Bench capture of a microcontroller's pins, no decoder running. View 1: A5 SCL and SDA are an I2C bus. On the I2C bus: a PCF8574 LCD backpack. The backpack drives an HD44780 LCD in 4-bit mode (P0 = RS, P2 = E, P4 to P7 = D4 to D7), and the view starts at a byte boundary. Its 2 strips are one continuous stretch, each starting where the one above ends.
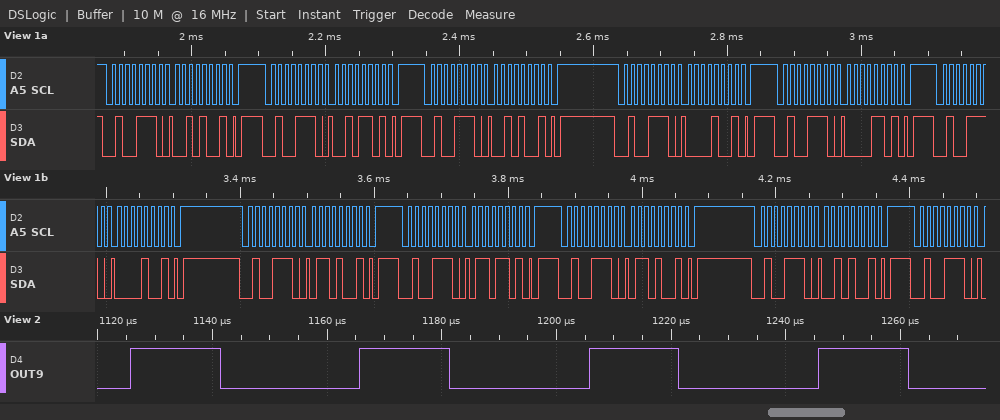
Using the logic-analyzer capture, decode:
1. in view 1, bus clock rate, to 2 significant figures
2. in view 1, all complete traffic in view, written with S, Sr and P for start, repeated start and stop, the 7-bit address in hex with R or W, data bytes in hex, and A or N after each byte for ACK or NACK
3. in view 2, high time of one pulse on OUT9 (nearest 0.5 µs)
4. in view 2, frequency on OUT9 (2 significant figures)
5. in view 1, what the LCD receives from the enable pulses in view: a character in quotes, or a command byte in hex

100 kHz
S 27W A 29 A P S 27W A 2D A P S 27W A 29 A P S 27W A 09 A P S 27W A 0D A P S 27W A 09 A P S 27W A 69 A P S 27W A 6D A P S 27W A 69 A P S 27W A 29 A P S 27W A
15.5 µs
25 kHz
' '
